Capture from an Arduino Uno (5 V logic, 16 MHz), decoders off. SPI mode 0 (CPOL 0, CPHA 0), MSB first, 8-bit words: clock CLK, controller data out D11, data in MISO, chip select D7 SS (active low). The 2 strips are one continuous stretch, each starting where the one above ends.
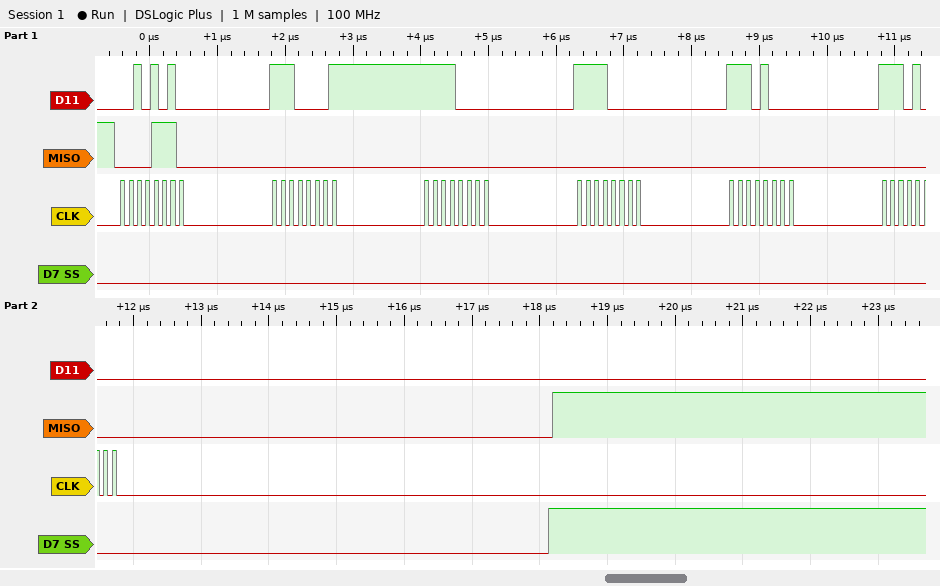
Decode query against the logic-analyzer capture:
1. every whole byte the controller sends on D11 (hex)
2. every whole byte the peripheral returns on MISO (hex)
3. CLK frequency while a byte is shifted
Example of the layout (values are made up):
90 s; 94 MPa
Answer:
0x2A 0xE1 0xF0 0xF0 0xE8 0xE8; 0x0E 0x00 0x00 0x00 0x00 0x00; 8 MHz
